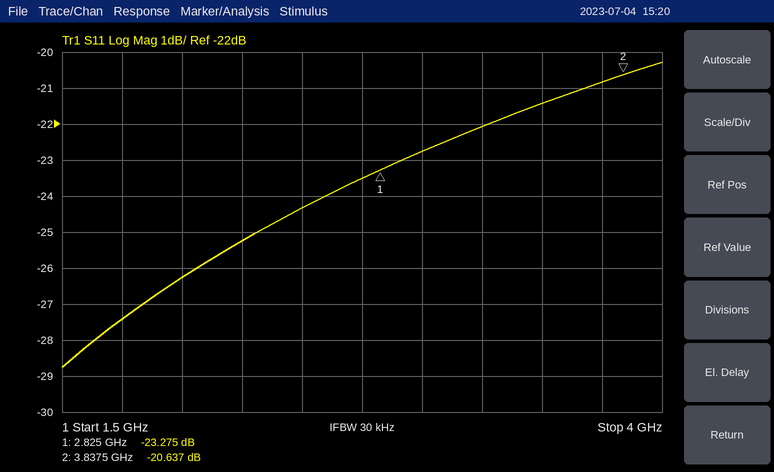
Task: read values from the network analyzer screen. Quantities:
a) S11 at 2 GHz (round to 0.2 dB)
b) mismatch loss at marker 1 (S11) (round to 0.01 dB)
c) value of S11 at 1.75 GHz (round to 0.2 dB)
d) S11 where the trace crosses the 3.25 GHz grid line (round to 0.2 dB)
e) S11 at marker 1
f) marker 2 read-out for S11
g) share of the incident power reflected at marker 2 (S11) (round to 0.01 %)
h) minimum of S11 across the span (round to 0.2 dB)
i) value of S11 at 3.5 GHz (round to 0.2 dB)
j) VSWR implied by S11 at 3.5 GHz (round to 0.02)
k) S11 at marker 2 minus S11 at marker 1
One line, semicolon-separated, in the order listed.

-26.2 dB; 0.02 dB; -27.4 dB; -22.0 dB; -23.275 dB; -20.637 dB; 0.86 %; -28.8 dB; -21.4 dB; 1.18; 2.638 dB
